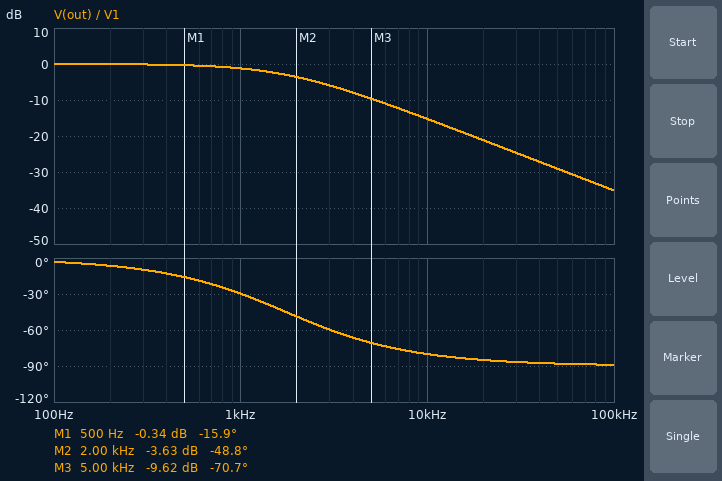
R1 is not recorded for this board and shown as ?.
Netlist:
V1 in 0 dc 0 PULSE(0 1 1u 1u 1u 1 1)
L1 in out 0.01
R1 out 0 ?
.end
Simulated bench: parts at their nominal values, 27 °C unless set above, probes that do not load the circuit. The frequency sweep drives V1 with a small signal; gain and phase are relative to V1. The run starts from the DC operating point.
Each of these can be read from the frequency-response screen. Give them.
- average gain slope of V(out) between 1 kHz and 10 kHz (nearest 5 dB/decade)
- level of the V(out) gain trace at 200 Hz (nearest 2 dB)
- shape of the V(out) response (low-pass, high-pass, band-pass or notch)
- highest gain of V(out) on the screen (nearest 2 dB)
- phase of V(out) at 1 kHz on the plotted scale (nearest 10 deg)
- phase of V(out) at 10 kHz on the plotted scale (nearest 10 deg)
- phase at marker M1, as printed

-15 dB/decade
0 dB
low-pass
0 dB
-30 deg
-80 deg
-15.9 deg
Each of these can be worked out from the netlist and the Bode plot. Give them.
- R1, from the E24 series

110 Ω
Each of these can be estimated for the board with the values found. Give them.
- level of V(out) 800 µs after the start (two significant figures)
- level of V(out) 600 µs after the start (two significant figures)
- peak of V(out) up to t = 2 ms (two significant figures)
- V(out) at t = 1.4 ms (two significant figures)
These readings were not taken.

1.0 V
1.0 V
1.0 V
1.0 V
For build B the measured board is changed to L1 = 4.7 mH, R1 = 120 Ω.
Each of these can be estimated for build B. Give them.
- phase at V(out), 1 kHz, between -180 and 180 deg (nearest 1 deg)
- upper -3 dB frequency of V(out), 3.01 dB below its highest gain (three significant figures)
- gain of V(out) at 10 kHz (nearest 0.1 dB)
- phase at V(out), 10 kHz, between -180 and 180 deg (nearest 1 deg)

-14 deg
4.06 kHz
-8.5 dB
-68 deg
